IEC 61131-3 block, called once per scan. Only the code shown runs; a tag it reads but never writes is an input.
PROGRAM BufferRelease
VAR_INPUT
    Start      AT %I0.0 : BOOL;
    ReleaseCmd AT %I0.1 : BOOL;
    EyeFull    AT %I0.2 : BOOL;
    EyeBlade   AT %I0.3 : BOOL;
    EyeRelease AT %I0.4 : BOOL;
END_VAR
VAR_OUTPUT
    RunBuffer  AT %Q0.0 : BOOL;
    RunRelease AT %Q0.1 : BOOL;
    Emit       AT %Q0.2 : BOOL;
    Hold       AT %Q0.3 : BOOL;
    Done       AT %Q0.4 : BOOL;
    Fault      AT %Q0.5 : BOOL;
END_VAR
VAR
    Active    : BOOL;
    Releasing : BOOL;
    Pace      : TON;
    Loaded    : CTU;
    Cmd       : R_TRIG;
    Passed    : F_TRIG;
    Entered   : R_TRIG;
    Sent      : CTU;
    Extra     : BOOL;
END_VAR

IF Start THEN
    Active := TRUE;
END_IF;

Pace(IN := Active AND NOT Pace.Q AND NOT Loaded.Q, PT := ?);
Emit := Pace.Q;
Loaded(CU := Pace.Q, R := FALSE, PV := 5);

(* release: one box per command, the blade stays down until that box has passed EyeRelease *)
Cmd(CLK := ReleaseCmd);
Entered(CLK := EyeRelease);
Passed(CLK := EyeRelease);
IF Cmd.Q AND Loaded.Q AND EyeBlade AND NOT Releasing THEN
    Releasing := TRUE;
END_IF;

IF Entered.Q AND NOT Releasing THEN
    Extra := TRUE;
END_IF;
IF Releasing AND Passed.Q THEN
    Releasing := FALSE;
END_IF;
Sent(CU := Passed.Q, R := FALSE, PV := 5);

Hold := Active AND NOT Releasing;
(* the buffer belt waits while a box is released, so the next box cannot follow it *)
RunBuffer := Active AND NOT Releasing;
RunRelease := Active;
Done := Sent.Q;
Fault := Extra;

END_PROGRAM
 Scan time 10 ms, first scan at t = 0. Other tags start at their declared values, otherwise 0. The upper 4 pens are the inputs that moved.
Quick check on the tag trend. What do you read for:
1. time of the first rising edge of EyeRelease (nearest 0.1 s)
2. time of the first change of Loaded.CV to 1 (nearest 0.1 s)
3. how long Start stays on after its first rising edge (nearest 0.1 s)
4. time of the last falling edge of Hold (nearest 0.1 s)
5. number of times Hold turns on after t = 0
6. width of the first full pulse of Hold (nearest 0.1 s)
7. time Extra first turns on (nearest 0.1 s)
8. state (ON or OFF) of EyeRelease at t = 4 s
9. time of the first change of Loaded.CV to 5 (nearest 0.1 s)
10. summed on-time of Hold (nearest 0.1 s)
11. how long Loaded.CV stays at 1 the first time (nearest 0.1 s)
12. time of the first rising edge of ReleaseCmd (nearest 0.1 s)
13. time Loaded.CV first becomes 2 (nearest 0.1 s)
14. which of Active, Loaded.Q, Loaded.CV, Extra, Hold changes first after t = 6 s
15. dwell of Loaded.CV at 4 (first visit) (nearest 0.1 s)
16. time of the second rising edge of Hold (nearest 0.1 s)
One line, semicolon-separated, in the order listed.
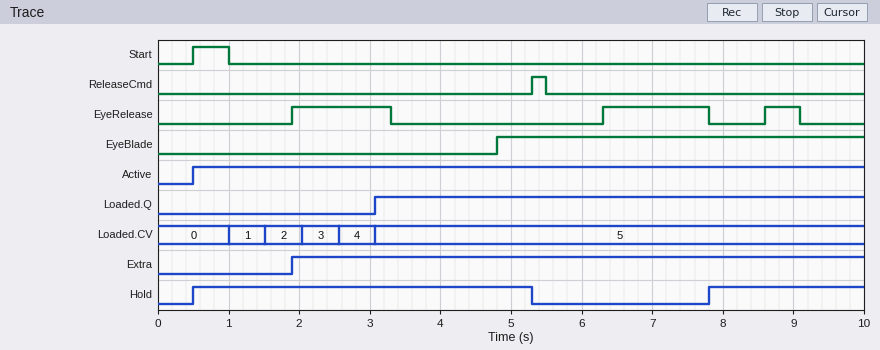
1.9 s; 1.0 s; 0.5 s; 5.3 s; 2; 4.8 s; 1.9 s; OFF; 3.1 s; 7.0 s; 0.5 s; 5.3 s; 1.5 s; Hold; 0.5 s; 7.8 s
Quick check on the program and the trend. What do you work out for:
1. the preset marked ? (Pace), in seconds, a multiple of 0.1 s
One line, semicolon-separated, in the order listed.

0.5 s
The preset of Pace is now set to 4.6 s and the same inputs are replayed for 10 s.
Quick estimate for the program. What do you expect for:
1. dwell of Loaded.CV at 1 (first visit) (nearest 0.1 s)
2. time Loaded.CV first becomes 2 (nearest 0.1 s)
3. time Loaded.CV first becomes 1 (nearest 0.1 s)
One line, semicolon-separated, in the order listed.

4.6 s; 9.7 s; 5.1 s
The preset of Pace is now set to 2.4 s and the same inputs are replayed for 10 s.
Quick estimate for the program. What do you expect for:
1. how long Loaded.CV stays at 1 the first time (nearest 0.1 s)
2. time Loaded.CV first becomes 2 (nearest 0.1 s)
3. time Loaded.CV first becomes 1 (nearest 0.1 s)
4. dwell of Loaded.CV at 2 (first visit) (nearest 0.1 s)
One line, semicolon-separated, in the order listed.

2.4 s; 5.3 s; 2.9 s; 2.4 s
